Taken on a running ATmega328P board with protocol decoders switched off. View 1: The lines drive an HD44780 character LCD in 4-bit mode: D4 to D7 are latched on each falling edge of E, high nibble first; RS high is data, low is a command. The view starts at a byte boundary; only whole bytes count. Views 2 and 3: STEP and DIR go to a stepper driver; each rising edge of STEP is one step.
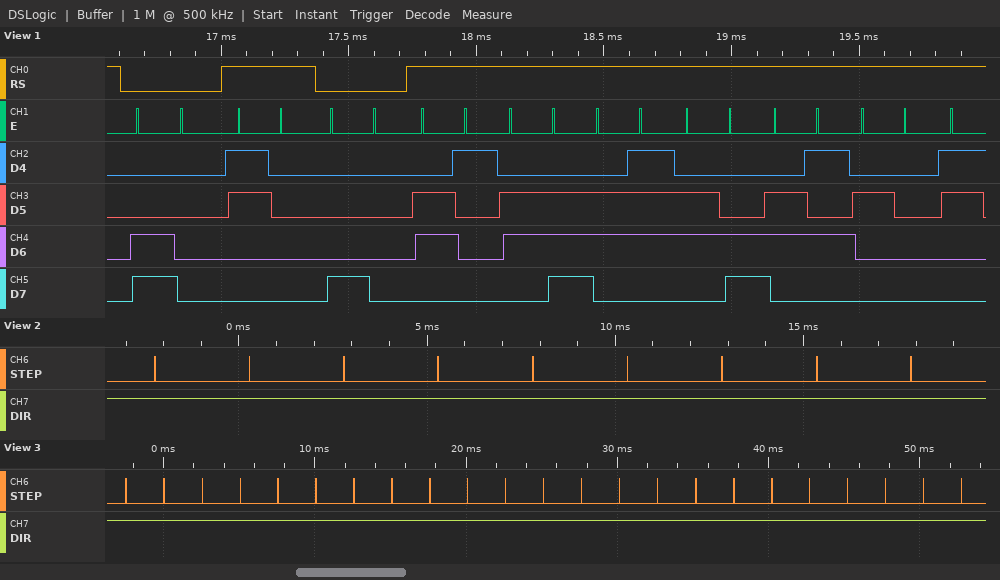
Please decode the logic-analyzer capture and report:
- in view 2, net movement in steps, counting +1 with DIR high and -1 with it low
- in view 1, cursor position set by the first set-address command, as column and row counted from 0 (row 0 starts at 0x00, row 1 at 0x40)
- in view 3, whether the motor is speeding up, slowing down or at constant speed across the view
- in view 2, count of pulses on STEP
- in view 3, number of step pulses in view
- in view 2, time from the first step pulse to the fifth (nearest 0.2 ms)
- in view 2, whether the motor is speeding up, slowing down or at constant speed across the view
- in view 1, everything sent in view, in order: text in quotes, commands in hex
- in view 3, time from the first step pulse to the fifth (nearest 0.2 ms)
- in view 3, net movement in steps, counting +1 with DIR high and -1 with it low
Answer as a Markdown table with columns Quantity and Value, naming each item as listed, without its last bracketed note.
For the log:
| Quantity | Value |
|---|---|
| in view 2, net movement in steps, counting +1 with DIR high and -1 with it low | +9 |
| in view 1, cursor position set by the first set-address command, as column and row counted from 0 | column 0, row 1 |
| in view 3, whether the motor is speeding up, slowing down or at constant speed across the view | constant speed |
| in view 2, count of pulses on STEP | 9 |
| in view 3, number of step pulses in view | 23 |
| in view 2, time from the first step pulse to the fifth | 10.0 ms |
| in view 2, whether the motor is speeding up, slowing down or at constant speed across the view | constant speed |
| in view 1, everything sent in view, in order: text in quotes, commands in hex | 0xC0 "0" 0x80 "angle " |
| in view 3, time from the first step pulse to the fifth | 10.0 ms |
| in view 3, net movement in steps, counting +1 with DIR high and -1 with it low | +23 |
